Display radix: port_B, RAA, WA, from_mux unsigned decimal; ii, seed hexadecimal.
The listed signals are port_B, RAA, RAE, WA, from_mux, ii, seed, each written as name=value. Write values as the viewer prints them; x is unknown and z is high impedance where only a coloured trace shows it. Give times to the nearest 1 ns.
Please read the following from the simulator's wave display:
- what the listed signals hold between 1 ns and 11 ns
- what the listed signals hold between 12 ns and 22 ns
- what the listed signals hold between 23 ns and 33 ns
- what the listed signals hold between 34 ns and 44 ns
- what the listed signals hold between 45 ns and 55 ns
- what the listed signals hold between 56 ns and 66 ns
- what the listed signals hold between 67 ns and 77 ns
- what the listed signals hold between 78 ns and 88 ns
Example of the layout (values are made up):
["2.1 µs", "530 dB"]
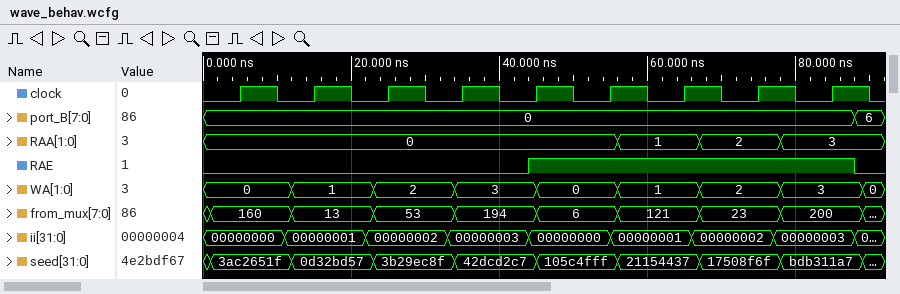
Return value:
["port_B=0, RAA=0, RAE=0, WA=0, from_mux=160, ii=00000000, seed=3ac2651f", "port_B=0, RAA=0, RAE=0, WA=1, from_mux=13, ii=00000001, seed=0d32bd57", "port_B=0, RAA=0, RAE=0, WA=2, from_mux=53, ii=00000002, seed=3b29ec8f", "port_B=0, RAA=0, RAE=0, WA=3, from_mux=194, ii=00000003, seed=42dcd2c7", "port_B=0, RAA=0, RAE=1, WA=0, from_mux=6, ii=00000000, seed=105c4fff", "port_B=0, RAA=1, RAE=1, WA=1, from_mux=121, ii=00000001, seed=21154437", "port_B=0, RAA=2, RAE=1, WA=2, from_mux=23, ii=00000002, seed=17508f6f", "port_B=0, RAA=3, RAE=1, WA=3, from_mux=200, ii=00000003, seed=bdb311a7"]
